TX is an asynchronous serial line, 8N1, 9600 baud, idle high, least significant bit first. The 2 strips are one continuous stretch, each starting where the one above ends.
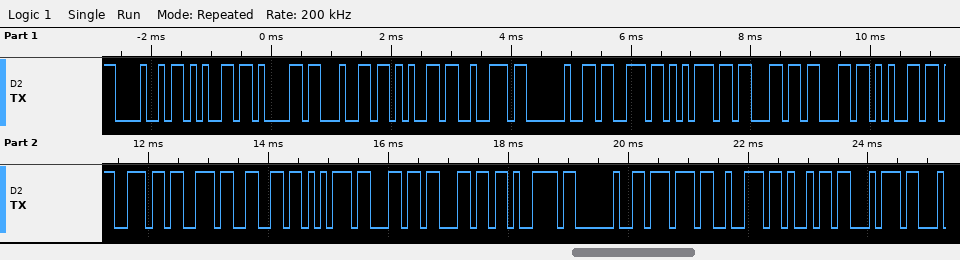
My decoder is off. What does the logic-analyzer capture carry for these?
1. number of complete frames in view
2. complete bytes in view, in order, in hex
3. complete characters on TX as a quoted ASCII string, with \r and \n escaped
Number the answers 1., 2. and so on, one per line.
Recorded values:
1. 24
2. 48 65 61 64 65 72 20 73 75 63 63 65 73 73 66 75 6C 6C 79 20 77 72 69 74
3. "Header successfully writ"
